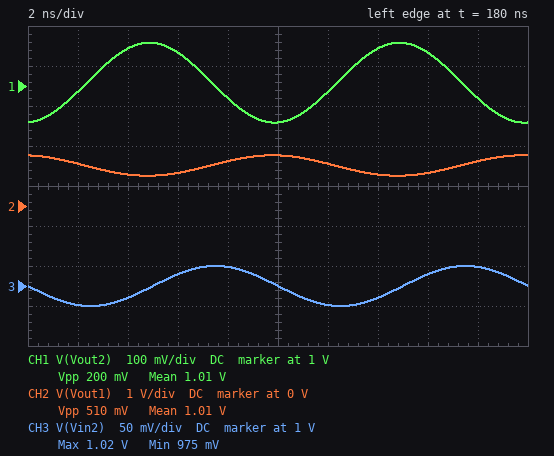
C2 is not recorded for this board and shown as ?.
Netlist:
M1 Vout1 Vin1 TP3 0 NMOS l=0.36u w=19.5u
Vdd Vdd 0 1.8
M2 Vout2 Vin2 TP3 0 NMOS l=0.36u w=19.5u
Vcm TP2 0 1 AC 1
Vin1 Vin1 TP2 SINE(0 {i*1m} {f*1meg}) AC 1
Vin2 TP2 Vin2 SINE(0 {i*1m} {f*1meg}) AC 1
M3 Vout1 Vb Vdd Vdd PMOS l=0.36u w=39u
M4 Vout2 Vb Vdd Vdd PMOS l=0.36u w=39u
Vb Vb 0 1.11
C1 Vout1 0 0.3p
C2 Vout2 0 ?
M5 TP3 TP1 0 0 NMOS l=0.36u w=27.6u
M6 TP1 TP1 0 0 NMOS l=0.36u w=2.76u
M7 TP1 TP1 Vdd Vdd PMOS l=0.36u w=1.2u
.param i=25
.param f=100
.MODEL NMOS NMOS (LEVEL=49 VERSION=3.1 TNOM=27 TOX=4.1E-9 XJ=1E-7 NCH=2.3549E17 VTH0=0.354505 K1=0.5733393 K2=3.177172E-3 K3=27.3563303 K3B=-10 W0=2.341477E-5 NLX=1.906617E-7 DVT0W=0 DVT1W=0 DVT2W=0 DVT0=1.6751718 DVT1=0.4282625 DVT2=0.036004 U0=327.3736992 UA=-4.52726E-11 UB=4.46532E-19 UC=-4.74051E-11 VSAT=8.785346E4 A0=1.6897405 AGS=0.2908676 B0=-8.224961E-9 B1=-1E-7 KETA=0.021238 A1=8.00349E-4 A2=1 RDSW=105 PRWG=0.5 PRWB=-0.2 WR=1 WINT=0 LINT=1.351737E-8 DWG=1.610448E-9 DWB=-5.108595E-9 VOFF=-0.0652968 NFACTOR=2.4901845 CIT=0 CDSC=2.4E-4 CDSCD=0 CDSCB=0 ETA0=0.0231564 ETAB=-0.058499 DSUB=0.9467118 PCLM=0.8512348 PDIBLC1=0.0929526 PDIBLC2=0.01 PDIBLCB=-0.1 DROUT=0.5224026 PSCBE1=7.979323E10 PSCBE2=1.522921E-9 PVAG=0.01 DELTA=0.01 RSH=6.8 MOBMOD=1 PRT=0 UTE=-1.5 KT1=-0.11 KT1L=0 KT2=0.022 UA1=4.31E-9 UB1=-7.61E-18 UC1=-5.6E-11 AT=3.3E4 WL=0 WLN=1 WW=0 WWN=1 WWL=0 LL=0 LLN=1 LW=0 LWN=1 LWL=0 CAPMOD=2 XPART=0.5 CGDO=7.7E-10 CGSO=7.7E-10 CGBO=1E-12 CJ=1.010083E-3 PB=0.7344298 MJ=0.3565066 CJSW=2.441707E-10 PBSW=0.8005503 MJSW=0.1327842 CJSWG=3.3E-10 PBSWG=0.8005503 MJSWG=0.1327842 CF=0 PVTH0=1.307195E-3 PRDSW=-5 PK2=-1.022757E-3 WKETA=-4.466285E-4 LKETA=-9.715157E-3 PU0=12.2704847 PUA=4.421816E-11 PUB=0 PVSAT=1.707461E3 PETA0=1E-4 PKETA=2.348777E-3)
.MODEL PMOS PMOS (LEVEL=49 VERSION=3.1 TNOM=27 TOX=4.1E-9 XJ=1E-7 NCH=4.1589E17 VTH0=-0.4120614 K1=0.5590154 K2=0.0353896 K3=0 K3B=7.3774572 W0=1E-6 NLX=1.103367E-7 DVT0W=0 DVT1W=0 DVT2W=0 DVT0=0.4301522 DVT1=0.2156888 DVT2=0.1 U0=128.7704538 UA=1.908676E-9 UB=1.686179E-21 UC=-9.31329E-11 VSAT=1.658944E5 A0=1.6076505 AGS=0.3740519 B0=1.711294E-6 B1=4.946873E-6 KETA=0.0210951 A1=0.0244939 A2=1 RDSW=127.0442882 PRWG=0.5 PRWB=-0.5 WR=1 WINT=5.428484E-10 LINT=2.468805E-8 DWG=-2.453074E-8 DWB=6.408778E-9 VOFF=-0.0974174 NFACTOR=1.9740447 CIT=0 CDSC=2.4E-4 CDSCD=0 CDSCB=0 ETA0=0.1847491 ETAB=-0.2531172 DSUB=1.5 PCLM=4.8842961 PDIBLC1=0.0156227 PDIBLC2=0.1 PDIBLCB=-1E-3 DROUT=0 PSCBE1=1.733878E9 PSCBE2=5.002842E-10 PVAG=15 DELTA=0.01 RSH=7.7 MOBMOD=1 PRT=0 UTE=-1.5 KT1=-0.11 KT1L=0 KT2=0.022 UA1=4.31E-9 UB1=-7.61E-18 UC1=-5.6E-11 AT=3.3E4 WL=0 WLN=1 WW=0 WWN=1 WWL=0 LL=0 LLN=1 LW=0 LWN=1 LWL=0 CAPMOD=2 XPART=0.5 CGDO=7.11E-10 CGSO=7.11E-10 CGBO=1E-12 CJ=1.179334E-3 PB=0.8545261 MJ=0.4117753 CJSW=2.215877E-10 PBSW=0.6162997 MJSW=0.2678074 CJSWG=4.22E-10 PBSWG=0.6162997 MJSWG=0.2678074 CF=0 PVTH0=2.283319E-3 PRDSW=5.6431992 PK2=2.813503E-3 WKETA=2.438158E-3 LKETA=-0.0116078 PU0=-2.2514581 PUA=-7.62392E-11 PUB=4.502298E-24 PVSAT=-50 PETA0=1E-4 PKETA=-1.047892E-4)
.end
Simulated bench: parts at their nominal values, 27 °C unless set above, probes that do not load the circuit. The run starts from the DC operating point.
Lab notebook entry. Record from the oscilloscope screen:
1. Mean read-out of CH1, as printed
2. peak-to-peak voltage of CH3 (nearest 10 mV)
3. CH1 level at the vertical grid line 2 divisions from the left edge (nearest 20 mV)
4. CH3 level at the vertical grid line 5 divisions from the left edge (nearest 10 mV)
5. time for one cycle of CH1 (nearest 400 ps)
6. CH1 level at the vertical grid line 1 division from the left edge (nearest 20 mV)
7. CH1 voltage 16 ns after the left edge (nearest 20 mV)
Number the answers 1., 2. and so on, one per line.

1. 1.01 V
2. 50 mV
3. 1.10 V
4. 1.00 V
5. 10.0 ns
6. 980 mV
7. 1.08 V
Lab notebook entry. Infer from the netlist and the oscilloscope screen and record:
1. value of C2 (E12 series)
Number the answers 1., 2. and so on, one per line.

1. 820 fF
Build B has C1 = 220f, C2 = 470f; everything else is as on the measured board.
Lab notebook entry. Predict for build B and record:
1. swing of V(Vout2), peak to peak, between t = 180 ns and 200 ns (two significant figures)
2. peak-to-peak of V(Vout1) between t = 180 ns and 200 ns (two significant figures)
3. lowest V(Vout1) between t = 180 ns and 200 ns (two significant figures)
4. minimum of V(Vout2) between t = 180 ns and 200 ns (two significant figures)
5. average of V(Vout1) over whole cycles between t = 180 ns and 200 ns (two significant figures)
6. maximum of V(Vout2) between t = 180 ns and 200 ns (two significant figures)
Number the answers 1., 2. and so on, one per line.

1. 330 mV
2. 660 mV
3. 680 mV
4. 840 mV
5. 1.0 V
6. 1.2 V
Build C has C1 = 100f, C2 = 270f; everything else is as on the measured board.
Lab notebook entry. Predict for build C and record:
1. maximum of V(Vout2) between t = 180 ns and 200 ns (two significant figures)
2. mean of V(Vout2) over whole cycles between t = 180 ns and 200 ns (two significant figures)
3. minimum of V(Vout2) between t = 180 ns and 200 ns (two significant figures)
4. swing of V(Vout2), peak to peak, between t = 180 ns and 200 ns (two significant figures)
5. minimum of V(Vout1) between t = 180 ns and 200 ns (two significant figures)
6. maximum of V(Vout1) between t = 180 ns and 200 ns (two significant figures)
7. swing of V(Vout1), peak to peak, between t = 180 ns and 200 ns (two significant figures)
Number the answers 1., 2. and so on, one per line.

1. 1.2 V
2. 970 mV
3. 720 mV
4. 500 mV
5. 450 mV
6. 1.6 V
7. 1.1 V
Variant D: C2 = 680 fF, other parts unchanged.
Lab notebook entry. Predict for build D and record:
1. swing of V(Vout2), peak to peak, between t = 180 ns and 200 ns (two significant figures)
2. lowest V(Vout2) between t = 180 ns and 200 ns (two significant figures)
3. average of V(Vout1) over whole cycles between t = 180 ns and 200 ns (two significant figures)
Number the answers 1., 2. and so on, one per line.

1. 240 mV
2. 890 mV
3. 1.0 V
